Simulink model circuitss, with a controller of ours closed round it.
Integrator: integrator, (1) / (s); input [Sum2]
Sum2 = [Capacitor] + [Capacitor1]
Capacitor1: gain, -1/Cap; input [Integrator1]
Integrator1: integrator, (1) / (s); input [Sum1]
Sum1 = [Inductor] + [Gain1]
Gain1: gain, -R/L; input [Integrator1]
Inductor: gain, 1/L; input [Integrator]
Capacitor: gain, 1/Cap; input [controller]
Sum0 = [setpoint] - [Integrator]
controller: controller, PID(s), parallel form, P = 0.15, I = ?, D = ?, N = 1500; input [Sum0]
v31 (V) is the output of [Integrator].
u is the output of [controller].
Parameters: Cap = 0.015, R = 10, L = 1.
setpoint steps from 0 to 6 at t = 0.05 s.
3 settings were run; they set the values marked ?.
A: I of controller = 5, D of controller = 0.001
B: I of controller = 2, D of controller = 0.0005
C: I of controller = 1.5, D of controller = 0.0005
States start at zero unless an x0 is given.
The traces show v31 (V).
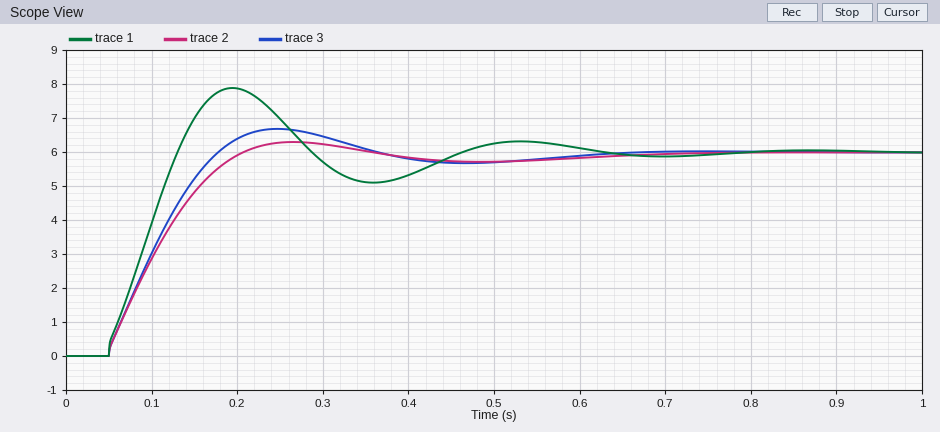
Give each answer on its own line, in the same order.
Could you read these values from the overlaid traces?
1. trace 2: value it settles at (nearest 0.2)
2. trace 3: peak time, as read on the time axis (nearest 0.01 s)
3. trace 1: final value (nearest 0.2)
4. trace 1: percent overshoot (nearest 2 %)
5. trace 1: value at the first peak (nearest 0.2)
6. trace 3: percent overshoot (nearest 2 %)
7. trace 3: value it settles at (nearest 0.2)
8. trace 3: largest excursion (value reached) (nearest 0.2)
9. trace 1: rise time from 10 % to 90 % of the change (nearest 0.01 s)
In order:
6.0
0.25 s
6.0
32 %
7.8
12 %
6.0
6.6
0.07 s
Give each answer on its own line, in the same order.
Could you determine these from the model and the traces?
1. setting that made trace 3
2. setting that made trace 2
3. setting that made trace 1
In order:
B
C
A
